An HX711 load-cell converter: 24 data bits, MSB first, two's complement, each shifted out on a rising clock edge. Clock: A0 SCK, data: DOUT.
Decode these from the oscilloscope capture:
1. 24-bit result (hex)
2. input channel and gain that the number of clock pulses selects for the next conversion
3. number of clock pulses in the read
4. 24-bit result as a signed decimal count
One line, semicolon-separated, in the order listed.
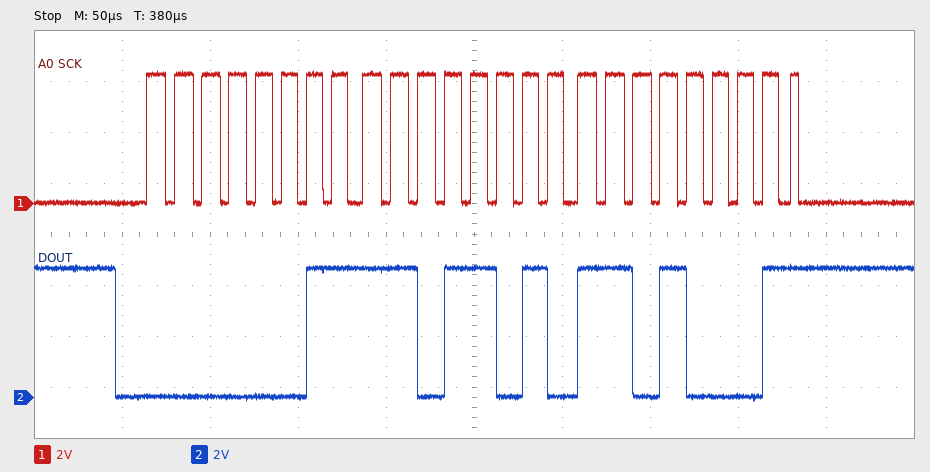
0x03DAD1; channel A, gain 128; 25; 252625
